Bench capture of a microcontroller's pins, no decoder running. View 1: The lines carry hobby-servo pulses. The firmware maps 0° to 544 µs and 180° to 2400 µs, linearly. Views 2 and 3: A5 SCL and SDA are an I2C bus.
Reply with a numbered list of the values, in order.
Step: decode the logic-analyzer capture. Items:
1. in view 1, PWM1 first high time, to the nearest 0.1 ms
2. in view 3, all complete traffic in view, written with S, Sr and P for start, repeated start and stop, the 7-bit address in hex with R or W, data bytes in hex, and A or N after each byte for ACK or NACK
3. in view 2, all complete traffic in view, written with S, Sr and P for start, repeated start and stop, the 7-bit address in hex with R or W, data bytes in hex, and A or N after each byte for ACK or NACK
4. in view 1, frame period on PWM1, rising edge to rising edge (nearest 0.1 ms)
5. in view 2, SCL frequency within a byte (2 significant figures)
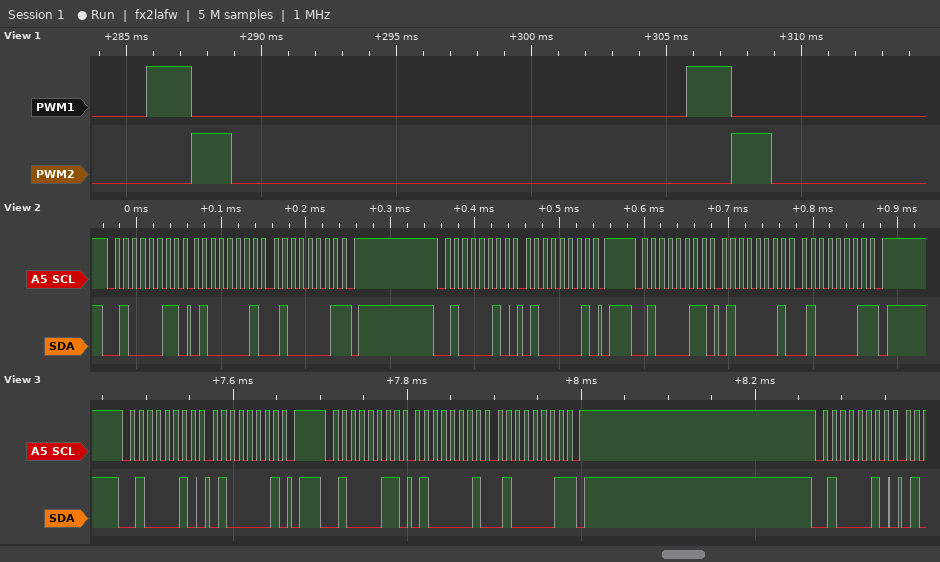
1. 1.7 ms
2. S 21W A 41 A P S 21R A 41 A 41 N P S 21W A
3. S 21R A 41 A 41 N P S 21W A 41 A P S 21R A 41 A 41 N P
4. 20.0 ms
5. 100 kHz
